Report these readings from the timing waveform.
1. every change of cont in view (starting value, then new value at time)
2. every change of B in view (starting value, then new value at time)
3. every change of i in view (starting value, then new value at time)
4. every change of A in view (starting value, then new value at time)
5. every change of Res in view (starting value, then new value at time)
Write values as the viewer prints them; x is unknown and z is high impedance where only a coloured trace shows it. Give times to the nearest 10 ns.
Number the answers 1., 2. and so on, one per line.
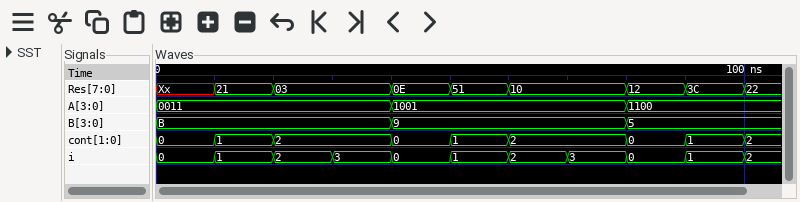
1. 0, 1 at 10 ns, 2 at 20 ns, 0 at 40 ns, 1 at 50 ns, 2 at 60 ns, 0 at 80 ns, 1 at 90 ns, 2 at 100 ns
2. B, 9 at 40 ns, 5 at 80 ns
3. 0, 1 at 10 ns, 2 at 20 ns, 3 at 30 ns, 0 at 40 ns, 1 at 50 ns, 2 at 60 ns, 3 at 70 ns, 0 at 80 ns, 1 at 90 ns, 2 at 100 ns
4. 0011, 1001 at 40 ns, 1100 at 80 ns
5. Xx, 21 at 10 ns, 03 at 20 ns, 0E at 40 ns, 51 at 50 ns, 10 at 60 ns, 12 at 80 ns, 3C at 90 ns, 22 at 100 ns
